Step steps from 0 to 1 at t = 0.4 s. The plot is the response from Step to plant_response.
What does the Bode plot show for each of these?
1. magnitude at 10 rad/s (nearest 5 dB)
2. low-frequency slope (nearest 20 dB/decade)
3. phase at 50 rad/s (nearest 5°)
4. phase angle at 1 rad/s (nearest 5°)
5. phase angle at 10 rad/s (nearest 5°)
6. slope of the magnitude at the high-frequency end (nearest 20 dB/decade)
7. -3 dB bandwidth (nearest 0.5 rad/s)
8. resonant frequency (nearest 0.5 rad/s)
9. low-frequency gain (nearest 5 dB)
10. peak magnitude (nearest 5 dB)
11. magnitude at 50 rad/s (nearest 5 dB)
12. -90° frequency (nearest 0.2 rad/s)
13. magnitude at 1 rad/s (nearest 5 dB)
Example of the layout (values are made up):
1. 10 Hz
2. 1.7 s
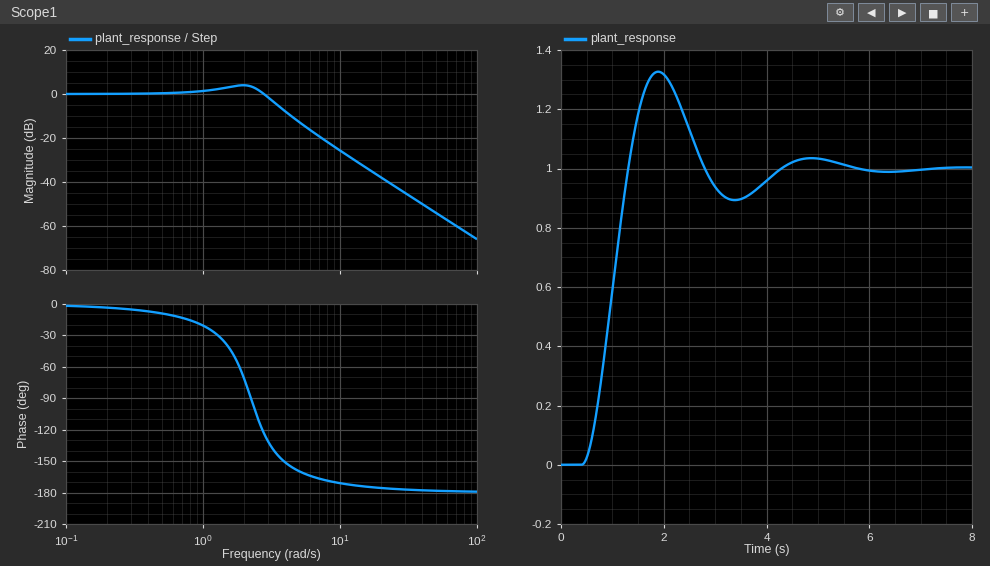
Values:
1. -25 dB
2. 0 dB/decade
3. -180°
4. -20°
5. -170°
6. -40 dB/decade
7. 3.0 rad/s
8. 2.0 rad/s
9. 0 dB
10. 5 dB
11. -55 dB
12. 2.2 rad/s
13. 0 dB
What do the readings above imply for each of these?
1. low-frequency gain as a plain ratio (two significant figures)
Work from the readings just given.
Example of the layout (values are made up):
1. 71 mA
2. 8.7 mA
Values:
1. 1.0
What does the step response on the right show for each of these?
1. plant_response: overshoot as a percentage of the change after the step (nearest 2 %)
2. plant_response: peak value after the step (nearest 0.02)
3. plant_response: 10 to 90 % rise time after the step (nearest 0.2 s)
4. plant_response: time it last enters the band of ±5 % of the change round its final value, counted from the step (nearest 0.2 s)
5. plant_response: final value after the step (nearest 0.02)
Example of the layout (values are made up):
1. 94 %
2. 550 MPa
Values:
1. 32 %
2. 1.32
3. 0.6 s
4. 3.6 s
5. 1.00
